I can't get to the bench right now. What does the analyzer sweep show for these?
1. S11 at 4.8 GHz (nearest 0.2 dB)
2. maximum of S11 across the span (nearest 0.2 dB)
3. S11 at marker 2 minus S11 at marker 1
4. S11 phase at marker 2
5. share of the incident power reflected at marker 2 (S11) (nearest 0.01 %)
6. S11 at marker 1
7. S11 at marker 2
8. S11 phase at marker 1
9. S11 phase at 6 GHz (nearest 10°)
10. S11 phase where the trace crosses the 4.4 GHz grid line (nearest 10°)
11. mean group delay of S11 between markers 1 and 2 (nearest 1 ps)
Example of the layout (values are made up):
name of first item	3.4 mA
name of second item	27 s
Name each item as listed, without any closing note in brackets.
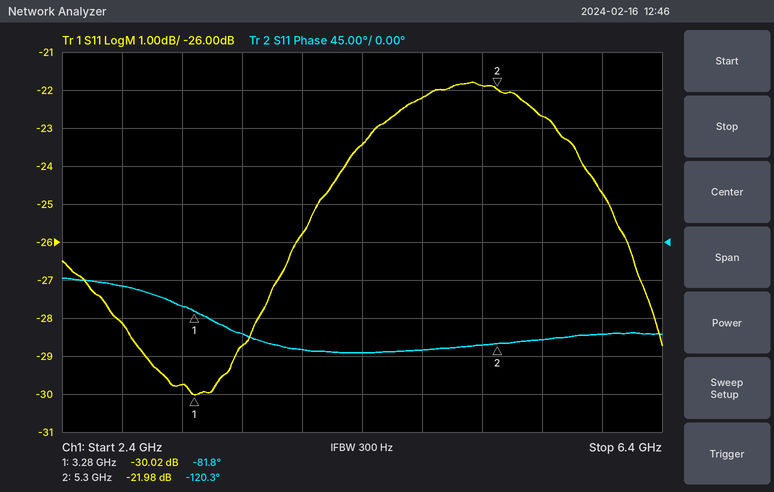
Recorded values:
S11 at 4.8 GHz	-22.2 dB
maximum of S11 across the span	-21.8 dB
S11 at marker 2 minus S11 at marker 1	8.04 dB
S11 phase at marker 2	-120.3°
share of the incident power reflected at marker 2 (S11)	0.63 %
S11 at marker 1	-30.02 dB
S11 at marker 2	-21.98 dB
S11 phase at marker 1	-81.8°
S11 phase at 6 GHz	-110°
S11 phase where the trace crosses the 4.4 GHz grid line	-130°
mean group delay of S11 between markers 1 and 2	53 ps
